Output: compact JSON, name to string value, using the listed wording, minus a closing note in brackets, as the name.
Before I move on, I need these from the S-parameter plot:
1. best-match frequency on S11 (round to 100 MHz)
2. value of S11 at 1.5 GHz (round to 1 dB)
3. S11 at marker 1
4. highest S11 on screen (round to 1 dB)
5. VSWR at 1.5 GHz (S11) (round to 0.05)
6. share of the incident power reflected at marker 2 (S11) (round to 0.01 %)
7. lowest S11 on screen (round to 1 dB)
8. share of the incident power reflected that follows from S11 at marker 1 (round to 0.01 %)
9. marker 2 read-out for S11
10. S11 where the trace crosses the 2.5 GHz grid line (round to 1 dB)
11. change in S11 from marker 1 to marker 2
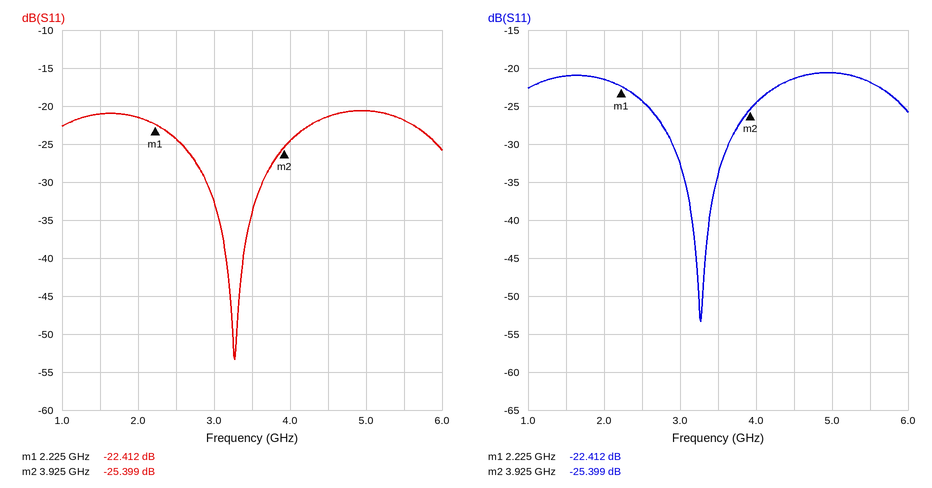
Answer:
{"best-match frequency on S11": "3.3 GHz", "value of S11 at 1.5 GHz": "-21 dB", "S11 at marker 1": "-22.412 dB", "highest S11 on screen": "-21 dB", "VSWR at 1.5 GHz (S11)": "1.20", "share of the incident power reflected at marker 2 (S11)": "0.29 %", "lowest S11 on screen": "-53 dB", "share of the incident power reflected that follows from S11 at marker 1": "0.57 %", "marker 2 read-out for S11": "-25.399 dB", "S11 where the trace crosses the 2.5 GHz grid line": "-24 dB", "change in S11 from marker 1 to marker 2": "-2.987 dB"}
